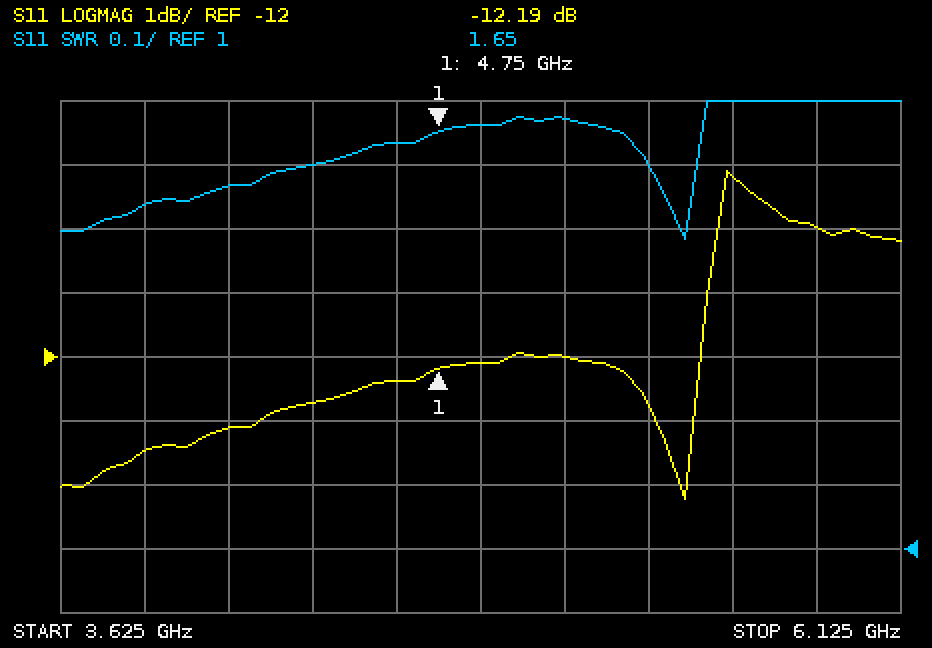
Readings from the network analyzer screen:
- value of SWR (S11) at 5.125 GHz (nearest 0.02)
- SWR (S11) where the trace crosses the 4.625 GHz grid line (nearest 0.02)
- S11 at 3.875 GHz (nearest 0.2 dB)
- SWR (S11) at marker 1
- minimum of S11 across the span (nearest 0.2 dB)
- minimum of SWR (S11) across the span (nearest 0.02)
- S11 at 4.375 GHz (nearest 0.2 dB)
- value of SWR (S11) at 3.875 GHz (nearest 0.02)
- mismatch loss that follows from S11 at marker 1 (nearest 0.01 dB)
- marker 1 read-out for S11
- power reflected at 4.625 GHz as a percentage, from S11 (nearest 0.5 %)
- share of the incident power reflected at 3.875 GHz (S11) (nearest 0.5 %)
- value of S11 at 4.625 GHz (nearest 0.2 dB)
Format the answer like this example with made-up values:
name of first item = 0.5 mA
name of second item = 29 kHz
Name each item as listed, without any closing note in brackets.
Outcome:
value of SWR (S11) at 5.125 GHz = 1.68
SWR (S11) where the trace crosses the 4.625 GHz grid line = 1.64
S11 at 3.875 GHz = -13.4 dB
SWR (S11) at marker 1 = 1.65
minimum of S11 across the span = -14.2 dB
minimum of SWR (S11) across the span = 1.48
S11 at 4.375 GHz = -12.8 dB
value of SWR (S11) at 3.875 GHz = 1.54
mismatch loss that follows from S11 at marker 1 = 0.27 dB
marker 1 read-out for S11 = -12.19 dB
power reflected at 4.625 GHz as a percentage, from S11 = 6.0 %
share of the incident power reflected at 3.875 GHz (S11) = 4.5 %
value of S11 at 4.625 GHz = -12.4 dB
